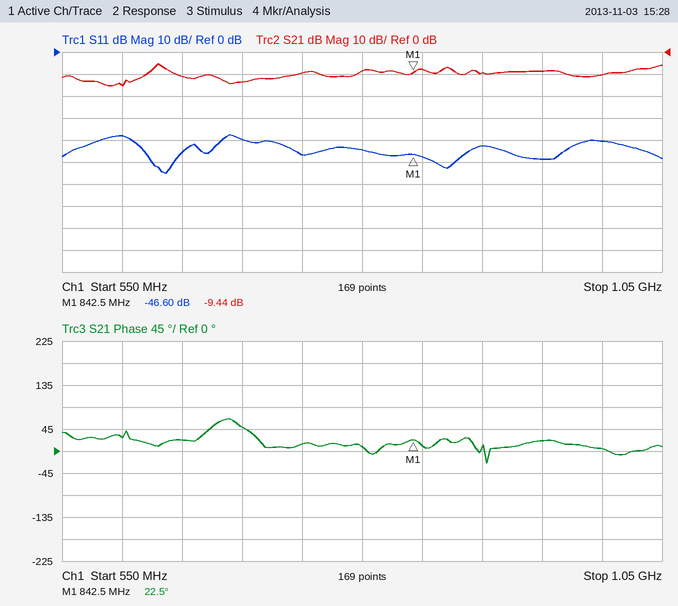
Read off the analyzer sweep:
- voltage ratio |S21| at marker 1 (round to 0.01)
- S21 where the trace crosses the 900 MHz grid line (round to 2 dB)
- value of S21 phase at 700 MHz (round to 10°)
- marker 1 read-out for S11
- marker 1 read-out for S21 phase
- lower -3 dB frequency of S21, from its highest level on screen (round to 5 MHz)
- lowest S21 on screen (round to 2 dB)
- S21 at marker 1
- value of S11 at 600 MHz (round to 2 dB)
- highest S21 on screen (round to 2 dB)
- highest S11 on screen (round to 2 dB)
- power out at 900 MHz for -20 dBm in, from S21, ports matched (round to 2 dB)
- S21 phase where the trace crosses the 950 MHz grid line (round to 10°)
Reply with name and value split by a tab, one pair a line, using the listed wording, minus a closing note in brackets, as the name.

voltage ratio |S21| at marker 1	0.34
S21 where the trace crosses the 900 MHz grid line	-10 dB
value of S21 phase at 700 MHz	50°
marker 1 read-out for S11	-46.60 dB
marker 1 read-out for S21 phase	22.5°
lower -3 dB frequency of S21, from its highest level on screen	625 MHz
lowest S21 on screen	-16 dB
S21 at marker 1	-9.44 dB
value of S11 at 600 MHz	-38 dB
highest S21 on screen	-6 dB
highest S11 on screen	-38 dB
power out at 900 MHz for -20 dBm in, from S21, ports matched	-30 dBm
S21 phase where the trace crosses the 950 MHz grid line	20°
